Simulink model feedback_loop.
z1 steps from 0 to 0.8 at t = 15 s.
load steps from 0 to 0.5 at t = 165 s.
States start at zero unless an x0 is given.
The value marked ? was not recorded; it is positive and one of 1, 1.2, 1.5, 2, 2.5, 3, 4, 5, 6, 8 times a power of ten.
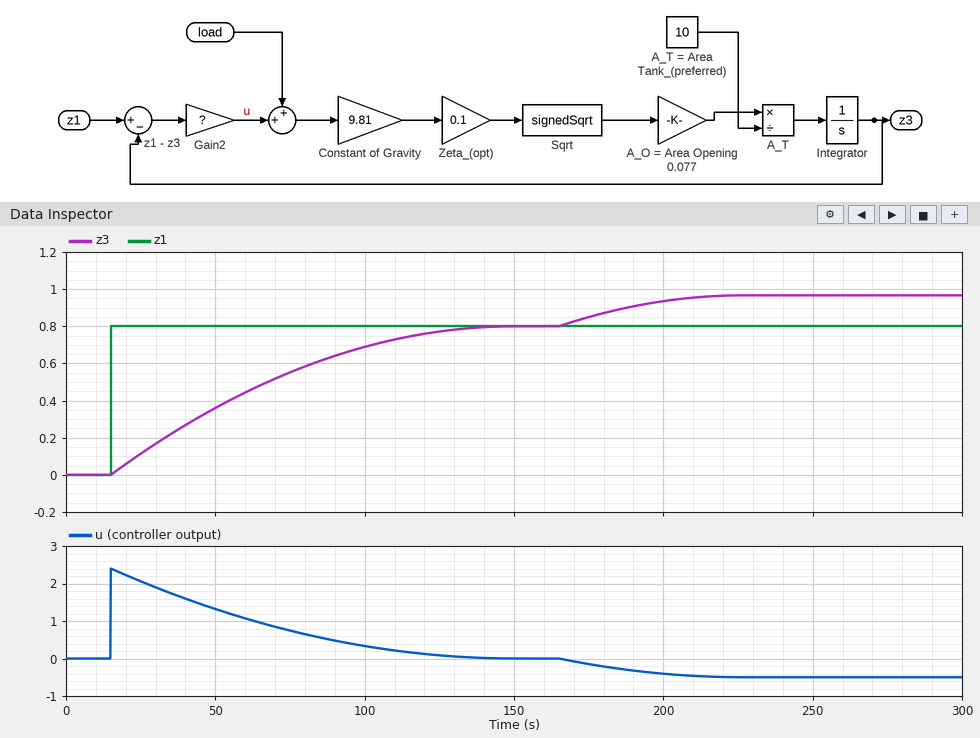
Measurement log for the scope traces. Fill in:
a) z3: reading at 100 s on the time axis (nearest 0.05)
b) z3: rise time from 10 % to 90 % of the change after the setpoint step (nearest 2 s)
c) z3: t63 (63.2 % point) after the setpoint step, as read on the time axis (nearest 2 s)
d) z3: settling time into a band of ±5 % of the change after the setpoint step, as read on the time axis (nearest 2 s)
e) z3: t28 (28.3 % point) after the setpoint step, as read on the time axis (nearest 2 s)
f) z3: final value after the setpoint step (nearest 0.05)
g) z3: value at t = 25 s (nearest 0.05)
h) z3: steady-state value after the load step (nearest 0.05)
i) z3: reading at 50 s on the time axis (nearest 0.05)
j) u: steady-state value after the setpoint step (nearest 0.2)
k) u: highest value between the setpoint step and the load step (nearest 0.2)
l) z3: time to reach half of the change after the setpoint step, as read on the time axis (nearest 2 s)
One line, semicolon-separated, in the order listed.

0.70; 86 s; 68 s; 120 s; 36 s; 0.80; 0.10; 0.95; 0.35; 0.0; 2.4; 54 s
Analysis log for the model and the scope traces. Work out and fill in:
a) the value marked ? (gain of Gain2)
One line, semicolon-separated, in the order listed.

3
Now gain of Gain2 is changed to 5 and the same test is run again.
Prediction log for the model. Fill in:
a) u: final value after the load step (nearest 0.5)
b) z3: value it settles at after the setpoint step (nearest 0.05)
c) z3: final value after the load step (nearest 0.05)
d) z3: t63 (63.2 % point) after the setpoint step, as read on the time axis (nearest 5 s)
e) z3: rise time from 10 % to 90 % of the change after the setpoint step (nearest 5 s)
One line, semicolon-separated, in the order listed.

-0.5; 0.80; 0.90; 55 s; 65 s
